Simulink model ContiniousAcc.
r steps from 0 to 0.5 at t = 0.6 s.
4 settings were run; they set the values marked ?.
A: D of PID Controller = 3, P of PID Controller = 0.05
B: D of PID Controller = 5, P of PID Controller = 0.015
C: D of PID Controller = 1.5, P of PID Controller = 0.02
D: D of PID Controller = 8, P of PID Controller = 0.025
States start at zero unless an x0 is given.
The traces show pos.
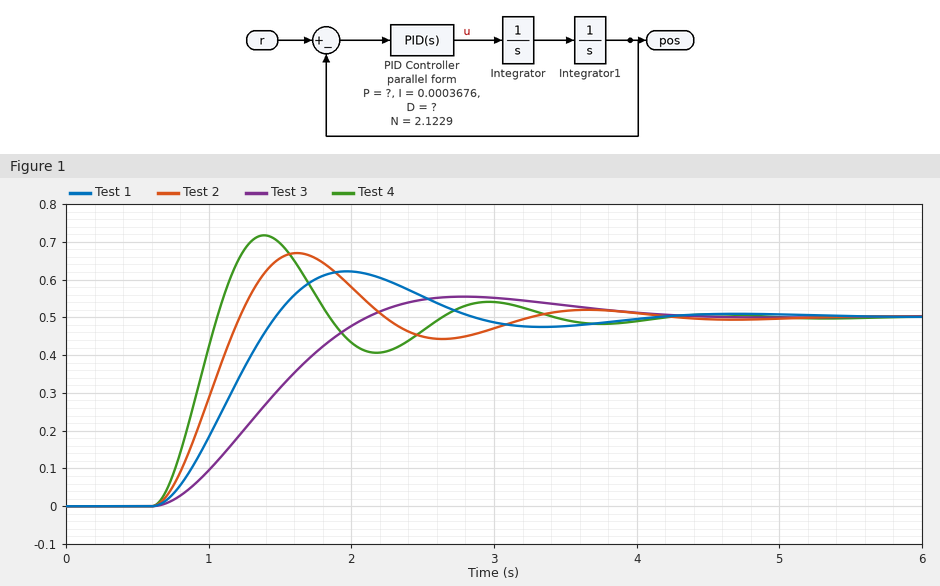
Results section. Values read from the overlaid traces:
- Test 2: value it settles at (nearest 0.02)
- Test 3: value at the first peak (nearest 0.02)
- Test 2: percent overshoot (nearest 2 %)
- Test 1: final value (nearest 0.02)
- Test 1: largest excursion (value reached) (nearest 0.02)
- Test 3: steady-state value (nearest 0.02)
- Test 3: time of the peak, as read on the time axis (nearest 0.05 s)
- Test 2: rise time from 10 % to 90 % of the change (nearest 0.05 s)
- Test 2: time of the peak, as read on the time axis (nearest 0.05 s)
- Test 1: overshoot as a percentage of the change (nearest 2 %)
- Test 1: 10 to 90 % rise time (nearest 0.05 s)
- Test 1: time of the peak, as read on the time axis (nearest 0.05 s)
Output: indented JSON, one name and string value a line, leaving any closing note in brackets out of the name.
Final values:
{
  "Test 2: value it settles at": "0.50",
  "Test 3: value at the first peak": "0.56",
  "Test 2: percent overshoot": "34 %",
  "Test 1: final value": "0.50",
  "Test 1: largest excursion (value reached)": "0.62",
  "Test 3: steady-state value": "0.50",
  "Test 3: time of the peak, as read on the time axis": "2.80 s",
  "Test 2: rise time from 10 % to 90 % of the change": "0.40 s",
  "Test 2: time of the peak, as read on the time axis": "1.60 s",
  "Test 1: overshoot as a percentage of the change": "24 %",
  "Test 1: 10 to 90 % rise time": "0.60 s",
  "Test 1: time of the peak, as read on the time axis": "1.95 s"
}
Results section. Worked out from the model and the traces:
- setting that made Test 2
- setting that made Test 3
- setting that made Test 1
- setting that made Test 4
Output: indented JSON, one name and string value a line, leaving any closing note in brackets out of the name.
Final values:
{
  "setting that made Test 2": "B",
  "setting that made Test 3": "C",
  "setting that made Test 1": "A",
  "setting that made Test 4": "D"
}
